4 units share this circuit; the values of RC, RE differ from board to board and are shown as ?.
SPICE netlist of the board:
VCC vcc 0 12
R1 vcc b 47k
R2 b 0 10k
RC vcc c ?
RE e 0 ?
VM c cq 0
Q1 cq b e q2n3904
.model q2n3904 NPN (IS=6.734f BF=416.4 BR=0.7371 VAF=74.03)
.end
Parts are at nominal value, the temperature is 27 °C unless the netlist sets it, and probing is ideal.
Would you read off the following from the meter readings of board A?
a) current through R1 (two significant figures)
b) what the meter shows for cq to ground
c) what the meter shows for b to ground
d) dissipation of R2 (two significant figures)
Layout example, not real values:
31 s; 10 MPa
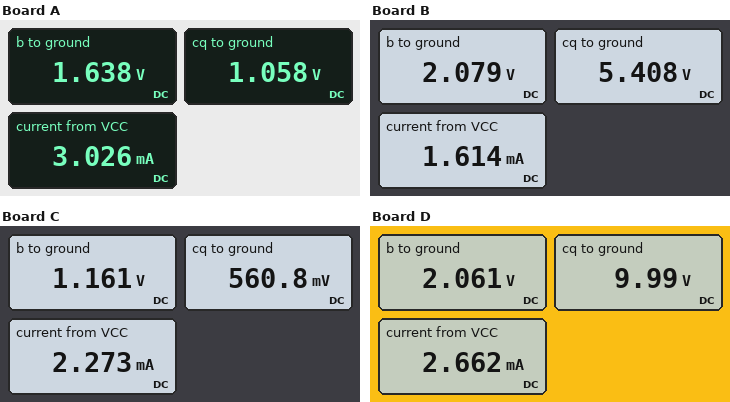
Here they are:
220 µA; 1.058 V; 1.638 V; 270 µW
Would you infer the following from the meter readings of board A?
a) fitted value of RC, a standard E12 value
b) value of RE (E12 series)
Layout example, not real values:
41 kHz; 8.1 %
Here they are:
3.9 kΩ; 330 Ω
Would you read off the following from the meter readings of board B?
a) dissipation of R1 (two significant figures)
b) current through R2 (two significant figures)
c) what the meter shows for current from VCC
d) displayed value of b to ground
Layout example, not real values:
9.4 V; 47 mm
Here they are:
2.1 mW; 210 µA; 1.614 mA; 2.079 V
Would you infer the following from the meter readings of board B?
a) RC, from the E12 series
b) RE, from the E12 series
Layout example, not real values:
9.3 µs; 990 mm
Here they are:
4.7 kΩ; 1 kΩ
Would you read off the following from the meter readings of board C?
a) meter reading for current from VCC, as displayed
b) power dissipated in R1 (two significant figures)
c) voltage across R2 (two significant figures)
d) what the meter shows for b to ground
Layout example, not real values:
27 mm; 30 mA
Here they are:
2.273 mA; 2.5 mW; 1.2 V; 1.161 V
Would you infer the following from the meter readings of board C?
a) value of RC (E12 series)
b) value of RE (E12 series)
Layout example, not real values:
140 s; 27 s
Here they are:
5.6 kΩ; 220 Ω
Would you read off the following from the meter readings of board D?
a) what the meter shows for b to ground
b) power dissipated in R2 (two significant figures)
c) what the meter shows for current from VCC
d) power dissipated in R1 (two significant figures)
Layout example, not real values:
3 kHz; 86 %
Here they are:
2.061 V; 420 µW; 2.662 mA; 2.1 mW
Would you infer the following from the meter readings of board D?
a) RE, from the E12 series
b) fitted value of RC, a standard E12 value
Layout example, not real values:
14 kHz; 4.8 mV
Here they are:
560 Ω; 820 Ω
